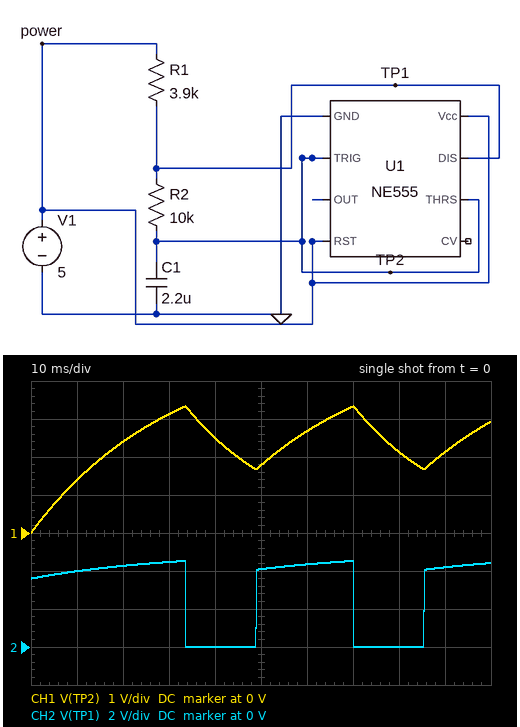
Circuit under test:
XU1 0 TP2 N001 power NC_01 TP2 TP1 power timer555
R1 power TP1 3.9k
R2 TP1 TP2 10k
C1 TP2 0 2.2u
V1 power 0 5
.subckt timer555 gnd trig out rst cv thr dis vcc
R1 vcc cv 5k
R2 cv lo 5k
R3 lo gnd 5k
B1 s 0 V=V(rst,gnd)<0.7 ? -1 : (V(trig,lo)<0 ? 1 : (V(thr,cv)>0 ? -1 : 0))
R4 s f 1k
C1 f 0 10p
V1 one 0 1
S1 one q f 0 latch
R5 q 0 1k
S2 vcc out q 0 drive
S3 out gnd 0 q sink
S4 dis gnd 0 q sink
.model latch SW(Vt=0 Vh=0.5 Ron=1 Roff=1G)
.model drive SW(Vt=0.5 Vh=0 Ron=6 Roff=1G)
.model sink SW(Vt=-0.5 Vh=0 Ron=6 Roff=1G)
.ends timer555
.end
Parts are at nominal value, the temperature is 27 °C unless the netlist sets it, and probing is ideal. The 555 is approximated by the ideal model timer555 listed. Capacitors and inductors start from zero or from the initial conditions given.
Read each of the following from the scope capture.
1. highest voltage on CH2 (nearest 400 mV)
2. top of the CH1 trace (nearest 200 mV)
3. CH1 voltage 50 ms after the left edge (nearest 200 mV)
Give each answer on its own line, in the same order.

4.4 V
3.4 V
1.8 V
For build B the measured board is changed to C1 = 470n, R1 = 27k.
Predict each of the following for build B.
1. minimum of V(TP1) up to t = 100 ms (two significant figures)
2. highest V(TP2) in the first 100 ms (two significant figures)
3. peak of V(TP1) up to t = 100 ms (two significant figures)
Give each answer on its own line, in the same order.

2.1 mV
3.3 V
3.8 V
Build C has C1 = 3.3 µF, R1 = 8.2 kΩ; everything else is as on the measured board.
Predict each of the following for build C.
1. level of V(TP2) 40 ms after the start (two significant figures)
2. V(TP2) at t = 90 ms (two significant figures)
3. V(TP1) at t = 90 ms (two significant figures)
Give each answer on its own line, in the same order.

2.4 V
1.7 V
3.5 V
